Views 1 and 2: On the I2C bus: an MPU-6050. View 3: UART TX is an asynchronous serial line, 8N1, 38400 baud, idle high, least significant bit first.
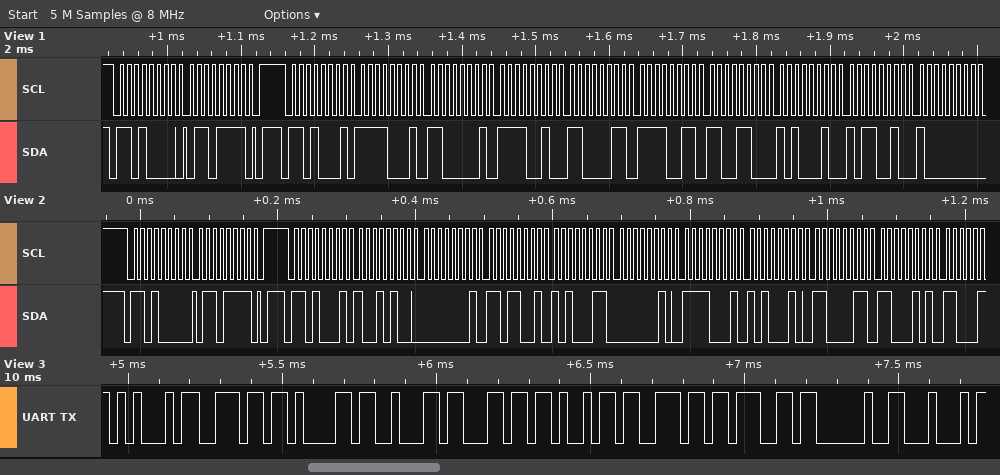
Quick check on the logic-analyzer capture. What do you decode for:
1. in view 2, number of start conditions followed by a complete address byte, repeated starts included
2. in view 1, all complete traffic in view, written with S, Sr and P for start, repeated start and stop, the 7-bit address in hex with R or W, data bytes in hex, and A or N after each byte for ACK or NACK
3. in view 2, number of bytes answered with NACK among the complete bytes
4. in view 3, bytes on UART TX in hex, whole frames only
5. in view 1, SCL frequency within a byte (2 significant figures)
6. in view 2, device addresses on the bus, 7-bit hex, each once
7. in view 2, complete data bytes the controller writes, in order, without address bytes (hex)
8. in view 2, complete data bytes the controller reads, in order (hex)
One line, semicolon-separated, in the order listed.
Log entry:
2; S 68W A 6F A P S 68R A F1 A C1 A F2 A C3 A F3 A CC A A2 A B2 A 80 A; 0; 45 6E 61 62 6C 69 6E 67 20 44; 100 kHz; 0x68; 6F; 94 01 D9 A3 02 F1 A2 C3 C5
